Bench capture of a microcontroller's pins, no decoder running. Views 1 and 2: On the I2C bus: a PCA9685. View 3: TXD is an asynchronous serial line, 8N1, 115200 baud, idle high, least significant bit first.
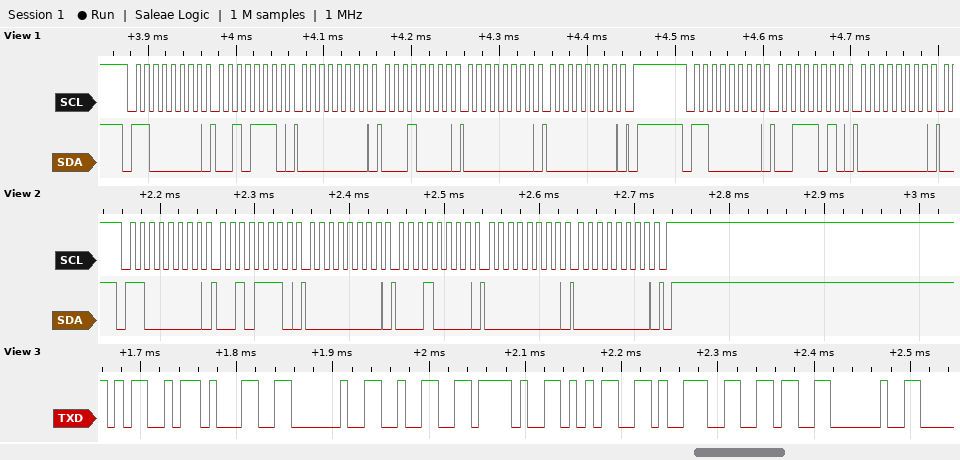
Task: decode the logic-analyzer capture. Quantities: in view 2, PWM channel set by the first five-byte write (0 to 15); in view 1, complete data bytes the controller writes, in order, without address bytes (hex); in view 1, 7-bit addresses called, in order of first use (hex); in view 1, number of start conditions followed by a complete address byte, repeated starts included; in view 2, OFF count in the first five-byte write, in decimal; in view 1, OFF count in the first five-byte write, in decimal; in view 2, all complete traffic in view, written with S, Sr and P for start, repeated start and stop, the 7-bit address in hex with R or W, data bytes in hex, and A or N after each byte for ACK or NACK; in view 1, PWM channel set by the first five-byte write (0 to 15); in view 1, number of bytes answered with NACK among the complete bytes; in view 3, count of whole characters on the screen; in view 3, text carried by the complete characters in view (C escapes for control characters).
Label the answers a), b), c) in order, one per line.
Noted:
a) 10
b) 2E 00 10 00 00 3A 00
c) 0x60
d) 2
e) 0
f) 0
g) S 60W A 2E A 00 A 10 A 00 A 00 A P
h) 10
i) 0
j) 9
k) "M1 2/596 "
